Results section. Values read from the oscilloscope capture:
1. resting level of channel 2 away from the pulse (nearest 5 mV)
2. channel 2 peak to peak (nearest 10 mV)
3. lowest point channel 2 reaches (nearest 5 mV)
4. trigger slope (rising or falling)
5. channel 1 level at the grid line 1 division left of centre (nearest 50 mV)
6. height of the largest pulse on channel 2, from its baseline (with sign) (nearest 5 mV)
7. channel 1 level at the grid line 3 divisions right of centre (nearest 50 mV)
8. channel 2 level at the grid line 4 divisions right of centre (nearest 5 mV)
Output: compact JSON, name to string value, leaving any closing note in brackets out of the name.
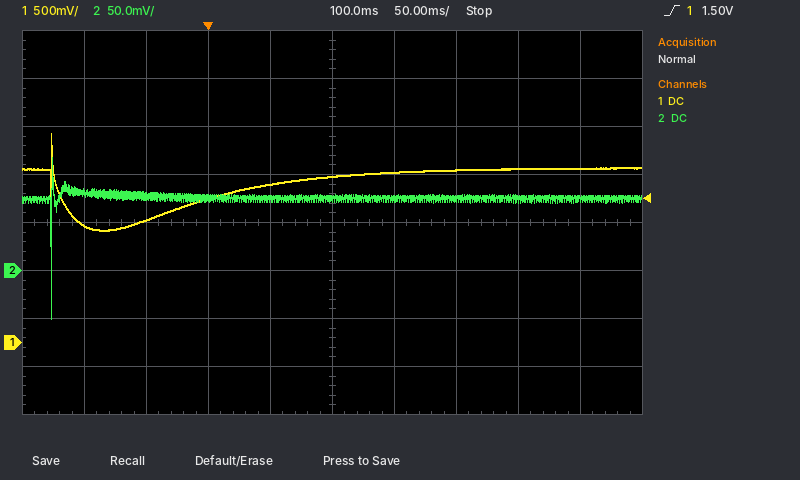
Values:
{"resting level of channel 2 away from the pulse": "75 mV", "channel 2 peak to peak": "170 mV", "lowest point channel 2 reaches": "-50 mV", "trigger slope": "rising", "channel 1 level at the grid line 1 division left of centre": "1.65 V", "height of the largest pulse on channel 2, from its baseline (with sign)": "-125 mV", "channel 1 level at the grid line 3 divisions right of centre": "1.80 V", "channel 2 level at the grid line 4 divisions right of centre": "75 mV"}
